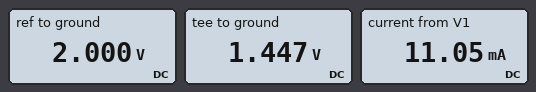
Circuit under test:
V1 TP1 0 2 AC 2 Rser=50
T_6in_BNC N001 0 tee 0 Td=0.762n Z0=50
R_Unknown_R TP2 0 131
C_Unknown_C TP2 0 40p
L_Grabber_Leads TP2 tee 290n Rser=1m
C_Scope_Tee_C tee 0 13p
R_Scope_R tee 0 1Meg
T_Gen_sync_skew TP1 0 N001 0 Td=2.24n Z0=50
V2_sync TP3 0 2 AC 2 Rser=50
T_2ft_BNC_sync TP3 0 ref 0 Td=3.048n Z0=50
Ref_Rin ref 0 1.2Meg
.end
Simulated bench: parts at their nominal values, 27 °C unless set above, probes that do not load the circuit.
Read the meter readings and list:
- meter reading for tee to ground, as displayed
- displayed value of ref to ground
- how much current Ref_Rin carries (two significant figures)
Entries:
1.447 V
2.000 V
1.7 µA
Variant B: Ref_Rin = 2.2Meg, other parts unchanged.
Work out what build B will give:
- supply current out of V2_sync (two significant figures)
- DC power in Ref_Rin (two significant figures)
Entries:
910 nA
1.8 µW
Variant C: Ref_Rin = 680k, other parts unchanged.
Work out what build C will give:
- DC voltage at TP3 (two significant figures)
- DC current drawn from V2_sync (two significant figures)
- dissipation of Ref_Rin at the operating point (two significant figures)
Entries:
2.0 V
2.9 µA
5.9 µW
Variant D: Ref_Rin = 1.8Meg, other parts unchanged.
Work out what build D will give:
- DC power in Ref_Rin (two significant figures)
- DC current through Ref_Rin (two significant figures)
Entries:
2.2 µW
1.1 µA
